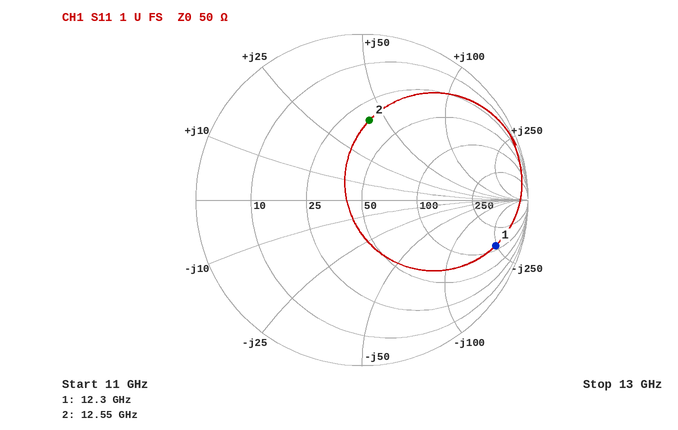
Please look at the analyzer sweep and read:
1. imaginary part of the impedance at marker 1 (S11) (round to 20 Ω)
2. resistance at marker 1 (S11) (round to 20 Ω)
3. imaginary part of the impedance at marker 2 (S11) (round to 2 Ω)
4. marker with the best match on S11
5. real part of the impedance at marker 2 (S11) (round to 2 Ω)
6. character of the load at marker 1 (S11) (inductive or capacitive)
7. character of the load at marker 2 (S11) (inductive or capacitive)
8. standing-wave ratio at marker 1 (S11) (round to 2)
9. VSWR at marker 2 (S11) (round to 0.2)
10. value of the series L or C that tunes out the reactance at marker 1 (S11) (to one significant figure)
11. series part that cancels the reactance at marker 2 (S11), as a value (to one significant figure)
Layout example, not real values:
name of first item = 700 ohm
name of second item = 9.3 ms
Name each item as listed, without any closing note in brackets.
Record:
imaginary part of the impedance at marker 1 (S11) = -240 Ω
resistance at marker 1 (S11) = 120 Ω
imaginary part of the impedance at marker 2 (S11) = +42 Ω
marker with the best match on S11 = marker 2
real part of the impedance at marker 2 (S11) = 34 Ω
character of the load at marker 1 (S11) = capacitive
character of the load at marker 2 (S11) = inductive
standing-wave ratio at marker 1 (S11) = 12
VSWR at marker 2 (S11) = 2.8
value of the series L or C that tunes out the reactance at marker 1 (S11) = 3 nH
series part that cancels the reactance at marker 2 (S11), as a value = 300 fF
